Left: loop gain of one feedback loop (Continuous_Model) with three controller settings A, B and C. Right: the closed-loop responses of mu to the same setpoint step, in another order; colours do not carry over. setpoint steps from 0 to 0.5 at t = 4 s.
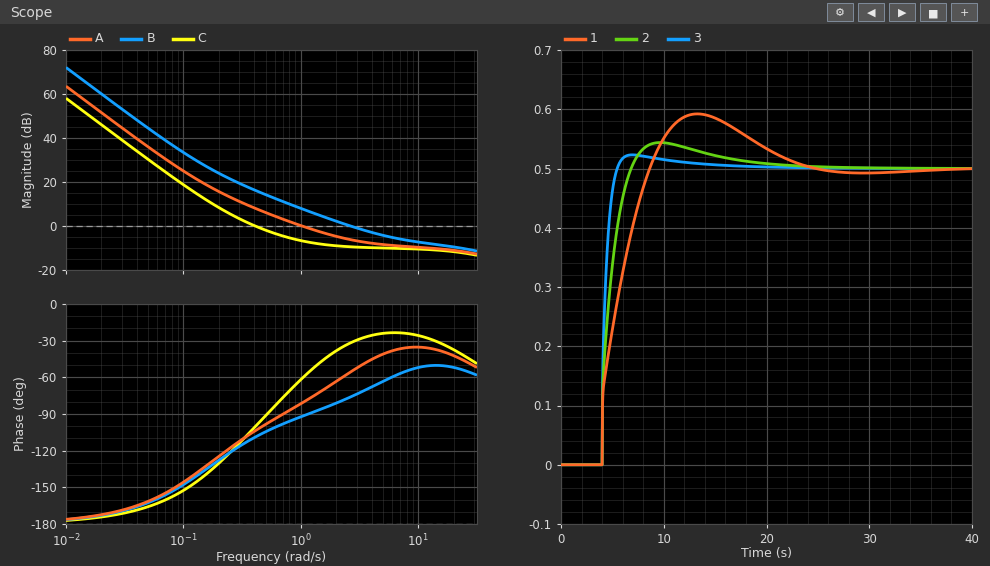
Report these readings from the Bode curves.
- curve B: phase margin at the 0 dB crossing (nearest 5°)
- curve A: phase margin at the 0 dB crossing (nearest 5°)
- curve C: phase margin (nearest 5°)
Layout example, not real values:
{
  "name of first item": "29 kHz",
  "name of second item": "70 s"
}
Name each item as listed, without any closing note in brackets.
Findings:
{
  "curve B: phase margin at the 0 dB crossing": "105°",
  "curve A: phase margin at the 0 dB crossing": "100°",
  "curve C: phase margin": "80°"
}
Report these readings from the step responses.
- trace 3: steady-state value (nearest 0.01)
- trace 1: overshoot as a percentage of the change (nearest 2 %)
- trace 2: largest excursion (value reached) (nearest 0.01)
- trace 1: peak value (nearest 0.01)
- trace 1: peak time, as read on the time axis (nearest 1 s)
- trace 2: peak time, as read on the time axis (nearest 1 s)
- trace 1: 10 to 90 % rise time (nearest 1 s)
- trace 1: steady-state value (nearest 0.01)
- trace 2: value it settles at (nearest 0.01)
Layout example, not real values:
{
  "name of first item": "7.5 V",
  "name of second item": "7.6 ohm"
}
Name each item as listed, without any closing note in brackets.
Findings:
{
  "trace 3: steady-state value": "0.50",
  "trace 1: overshoot as a percentage of the change": "18 %",
  "trace 2: largest excursion (value reached)": "0.54",
  "trace 1: peak value": "0.59",
  "trace 1: peak time, as read on the time axis": "13 s",
  "trace 2: peak time, as read on the time axis": "10 s",
  "trace 1: 10 to 90 % rise time": "4 s",
  "trace 1: steady-state value": "0.50",
  "trace 2: value it settles at": "0.50"
}
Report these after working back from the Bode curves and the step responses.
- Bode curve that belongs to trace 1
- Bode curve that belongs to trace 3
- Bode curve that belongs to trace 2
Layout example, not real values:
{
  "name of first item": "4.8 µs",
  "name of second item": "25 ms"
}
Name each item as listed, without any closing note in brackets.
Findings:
{
  "Bode curve that belongs to trace 1": "C",
  "Bode curve that belongs to trace 3": "B",
  "Bode curve that belongs to trace 2": "A"
}
